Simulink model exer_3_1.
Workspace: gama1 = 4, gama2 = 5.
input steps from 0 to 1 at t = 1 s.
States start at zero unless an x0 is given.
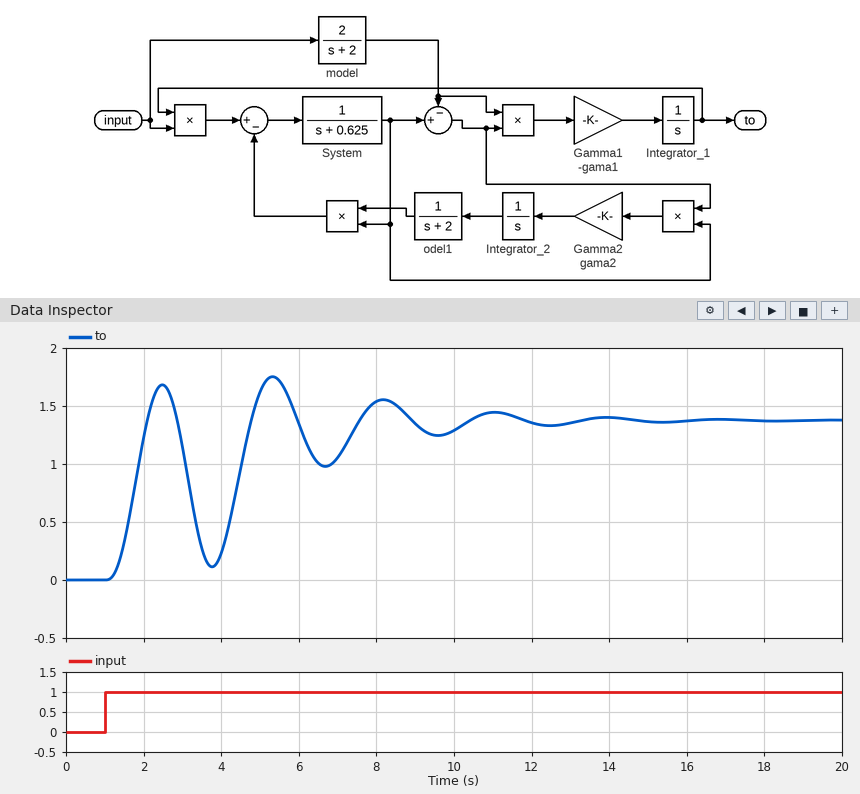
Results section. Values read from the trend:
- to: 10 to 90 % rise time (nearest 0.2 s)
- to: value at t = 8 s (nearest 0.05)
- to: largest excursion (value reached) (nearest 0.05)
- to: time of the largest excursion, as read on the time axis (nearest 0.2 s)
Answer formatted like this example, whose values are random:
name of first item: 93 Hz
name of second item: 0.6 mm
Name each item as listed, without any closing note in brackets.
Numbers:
to: 10 to 90 % rise time: 0.6 s
to: value at t = 8 s: 1.55
to: largest excursion (value reached): 1.75
to: time of the largest excursion, as read on the time axis: 5.4 s
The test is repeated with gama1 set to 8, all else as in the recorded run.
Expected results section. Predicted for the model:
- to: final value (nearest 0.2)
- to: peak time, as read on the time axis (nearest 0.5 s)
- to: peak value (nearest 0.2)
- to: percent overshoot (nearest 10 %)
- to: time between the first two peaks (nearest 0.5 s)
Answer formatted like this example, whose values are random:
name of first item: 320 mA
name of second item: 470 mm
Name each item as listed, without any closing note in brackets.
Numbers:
to: final value: 1.2
to: peak time, as read on the time axis: 2.0 s
to: peak value: 2.0
to: percent overshoot: 60 %
to: time between the first two peaks: 2.0 s
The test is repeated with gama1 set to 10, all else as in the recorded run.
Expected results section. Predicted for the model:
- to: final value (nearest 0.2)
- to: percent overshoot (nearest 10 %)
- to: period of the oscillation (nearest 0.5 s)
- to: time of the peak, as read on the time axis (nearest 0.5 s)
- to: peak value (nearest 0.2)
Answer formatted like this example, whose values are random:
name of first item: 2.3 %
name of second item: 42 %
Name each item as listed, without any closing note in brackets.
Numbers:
to: final value: 1.2
to: percent overshoot: 80 %
to: period of the oscillation: 2.0 s
to: time of the peak, as read on the time axis: 2.0 s
to: peak value: 2.2
